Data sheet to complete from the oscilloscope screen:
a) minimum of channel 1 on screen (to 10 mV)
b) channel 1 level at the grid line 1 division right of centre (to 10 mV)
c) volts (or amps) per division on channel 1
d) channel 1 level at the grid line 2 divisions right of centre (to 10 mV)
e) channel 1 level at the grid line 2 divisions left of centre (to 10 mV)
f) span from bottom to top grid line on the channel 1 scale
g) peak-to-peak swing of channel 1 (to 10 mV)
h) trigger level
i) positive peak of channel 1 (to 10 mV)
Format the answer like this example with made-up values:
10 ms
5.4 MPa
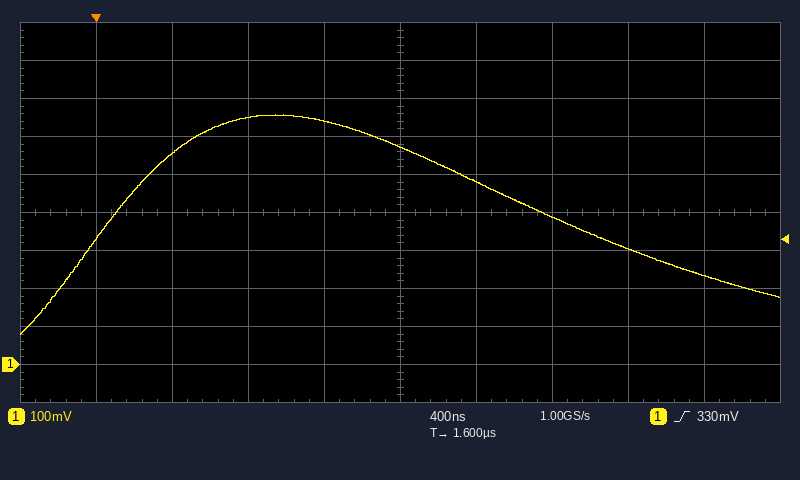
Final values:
80 mV
480 mV
100 mV
390 mV
650 mV
1 V
580 mV
330 mV
660 mV
